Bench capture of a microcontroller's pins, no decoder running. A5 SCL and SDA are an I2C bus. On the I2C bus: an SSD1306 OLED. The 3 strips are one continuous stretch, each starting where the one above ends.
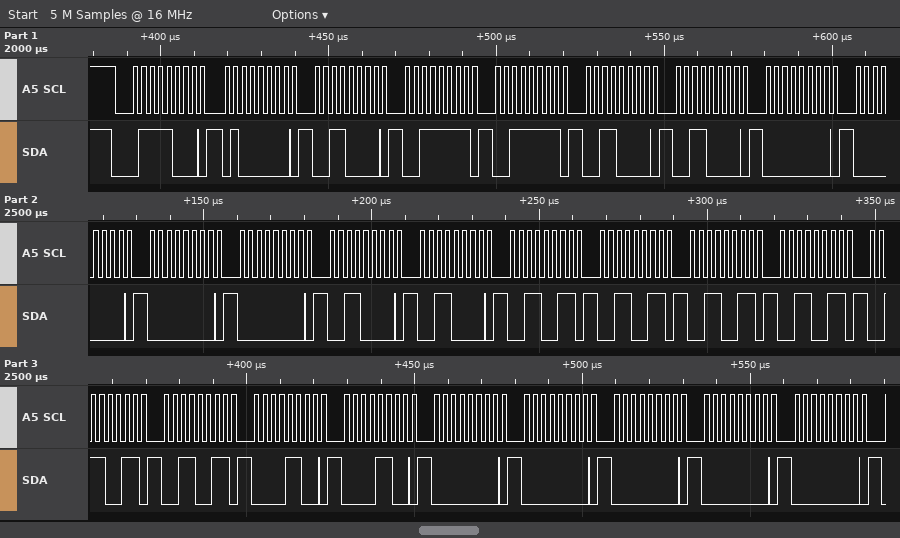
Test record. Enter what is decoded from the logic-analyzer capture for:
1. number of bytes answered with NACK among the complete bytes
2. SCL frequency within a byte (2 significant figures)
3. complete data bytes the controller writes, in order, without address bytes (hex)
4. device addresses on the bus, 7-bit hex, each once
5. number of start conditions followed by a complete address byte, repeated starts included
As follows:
0
400 kHz
40 30 3F 3F 30 30 00 00 00 00 30 30 33 33 33 33 33 33 0C 0C 00 00 00 00 00
0x3C
1
